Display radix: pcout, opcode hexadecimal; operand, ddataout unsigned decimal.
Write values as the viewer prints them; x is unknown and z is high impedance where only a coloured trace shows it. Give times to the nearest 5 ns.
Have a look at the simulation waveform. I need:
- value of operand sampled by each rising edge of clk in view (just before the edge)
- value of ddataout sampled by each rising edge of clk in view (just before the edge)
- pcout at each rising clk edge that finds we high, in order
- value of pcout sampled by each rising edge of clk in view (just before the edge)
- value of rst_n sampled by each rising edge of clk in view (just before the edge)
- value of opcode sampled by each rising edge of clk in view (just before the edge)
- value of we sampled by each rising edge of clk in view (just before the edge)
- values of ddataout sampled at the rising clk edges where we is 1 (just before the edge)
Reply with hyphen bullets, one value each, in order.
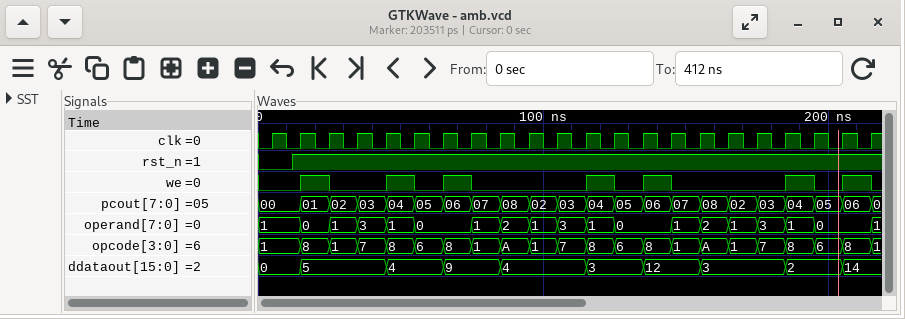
- 1, 1, 0, 1, 3, 1, 0, 0, 1, 2, 1, 3, 1, 0, 0, 1, 2, 1, 3, 1, 0, 0
- 0, 0, 5, 5, 5, 4, 4, 9, 9, 4, 4, 4, 3, 3, 12, 12, 3, 3, 3, 2, 2, 14
- 01, 04, 06, 04, 06, 04, 06
- 00, 00, 01, 02, 03, 04, 05, 06, 07, 08, 02, 03, 04, 05, 06, 07, 08, 02, 03, 04, 05, 06
- 0 1 1 1 1 1 1 1 1 1 1 1 1 1 1 1 1 1 1 1 1 1
- 1, 1, 8, 1, 7, 8, 6, 8, 1, A, 1, 7, 8, 6, 8, 1, A, 1, 7, 8, 6, 8
- 0 0 1 0 0 1 0 1 0 0 0 0 1 0 1 0 0 0 0 1 0 1
- 5, 4, 9, 3, 12, 2, 14
